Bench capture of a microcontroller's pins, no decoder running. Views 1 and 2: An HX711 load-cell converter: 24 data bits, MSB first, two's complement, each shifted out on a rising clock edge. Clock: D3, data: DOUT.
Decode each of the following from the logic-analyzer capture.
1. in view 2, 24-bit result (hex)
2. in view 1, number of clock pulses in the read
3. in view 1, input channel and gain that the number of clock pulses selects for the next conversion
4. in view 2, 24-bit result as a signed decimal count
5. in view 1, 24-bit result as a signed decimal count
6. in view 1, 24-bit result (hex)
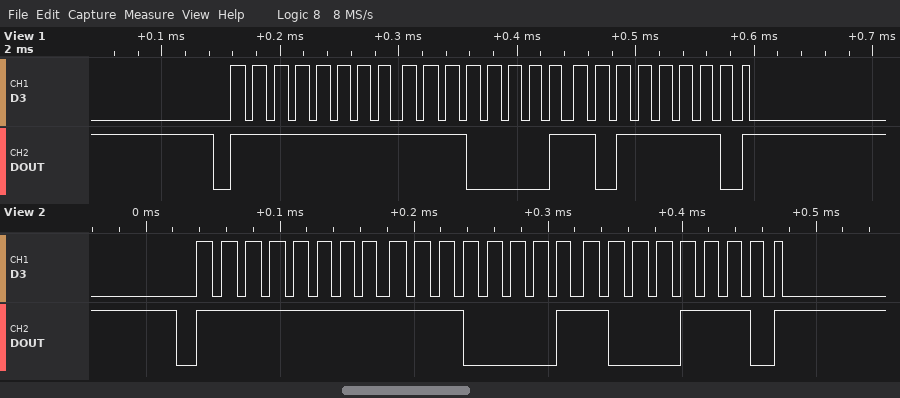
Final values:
0xFFE18E
25
channel A, gain 128
-7794
-7746
0xFFE1BE
